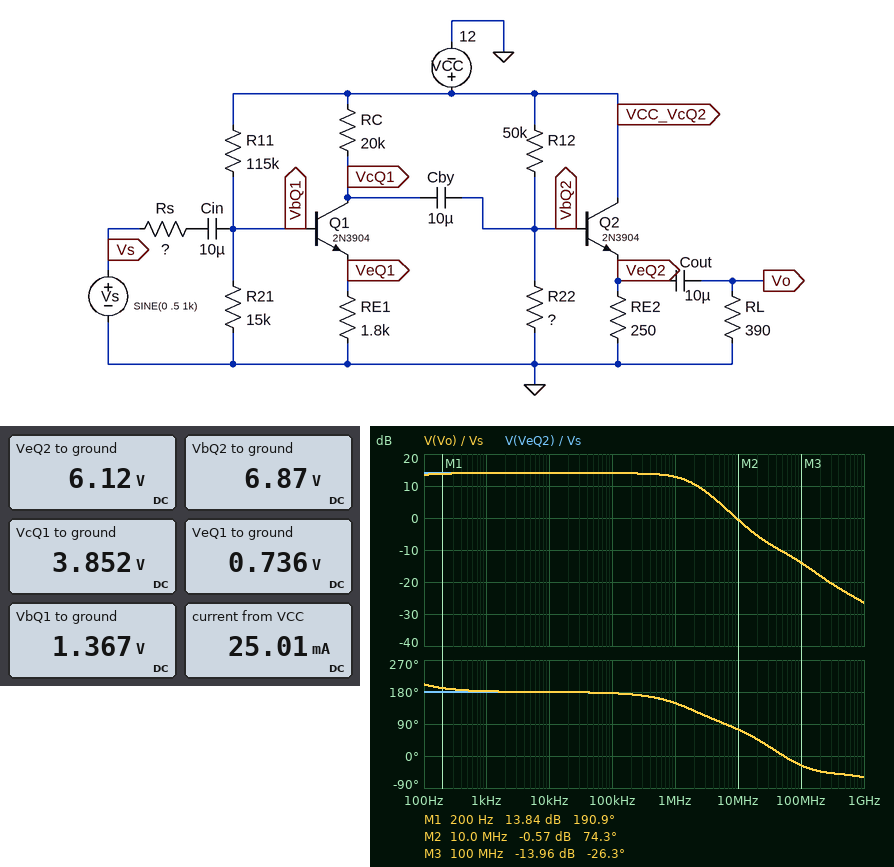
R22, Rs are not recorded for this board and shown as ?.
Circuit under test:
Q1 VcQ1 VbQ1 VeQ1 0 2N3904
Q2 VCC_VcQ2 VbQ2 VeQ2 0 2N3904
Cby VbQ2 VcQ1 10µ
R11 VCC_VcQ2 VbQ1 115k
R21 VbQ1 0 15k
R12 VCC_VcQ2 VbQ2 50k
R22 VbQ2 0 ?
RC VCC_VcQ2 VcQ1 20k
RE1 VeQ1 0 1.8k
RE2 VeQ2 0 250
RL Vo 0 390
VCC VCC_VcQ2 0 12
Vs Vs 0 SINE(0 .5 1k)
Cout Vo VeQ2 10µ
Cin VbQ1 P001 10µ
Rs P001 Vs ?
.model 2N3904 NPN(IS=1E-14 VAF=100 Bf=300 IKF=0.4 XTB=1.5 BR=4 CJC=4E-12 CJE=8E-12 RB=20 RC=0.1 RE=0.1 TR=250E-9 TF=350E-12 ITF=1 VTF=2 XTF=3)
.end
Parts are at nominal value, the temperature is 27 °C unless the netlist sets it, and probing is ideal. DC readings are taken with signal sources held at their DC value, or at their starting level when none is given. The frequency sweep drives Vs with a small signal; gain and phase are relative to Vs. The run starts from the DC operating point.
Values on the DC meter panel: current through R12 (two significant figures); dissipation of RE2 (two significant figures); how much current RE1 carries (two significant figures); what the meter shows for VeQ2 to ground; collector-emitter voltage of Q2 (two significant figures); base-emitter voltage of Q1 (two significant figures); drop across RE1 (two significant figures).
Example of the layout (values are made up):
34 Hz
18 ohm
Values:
100 µA
150 mW
410 µA
6.12 V
5.9 V
630 mV
740 mV
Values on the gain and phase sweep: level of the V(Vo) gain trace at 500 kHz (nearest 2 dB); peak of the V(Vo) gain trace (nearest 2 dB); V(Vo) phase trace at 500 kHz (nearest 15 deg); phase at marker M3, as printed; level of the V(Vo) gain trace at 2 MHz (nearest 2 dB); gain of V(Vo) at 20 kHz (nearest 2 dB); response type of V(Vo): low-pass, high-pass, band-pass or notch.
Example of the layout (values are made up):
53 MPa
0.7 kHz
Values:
14 dB
14 dB
165 deg
-26.3 deg
10 dB
14 dB
low-pass
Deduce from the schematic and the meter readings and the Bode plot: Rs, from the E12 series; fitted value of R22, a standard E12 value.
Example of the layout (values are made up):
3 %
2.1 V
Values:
1.2 kΩ
330 kΩ
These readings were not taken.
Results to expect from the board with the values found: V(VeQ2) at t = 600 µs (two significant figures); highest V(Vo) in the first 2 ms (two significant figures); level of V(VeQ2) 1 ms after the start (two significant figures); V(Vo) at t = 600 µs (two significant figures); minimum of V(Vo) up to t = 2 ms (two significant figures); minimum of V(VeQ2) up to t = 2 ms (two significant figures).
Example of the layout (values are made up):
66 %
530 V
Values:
7.6 V
2.5 V
6.1 V
1.6 V
-2.4 V
3.6 V
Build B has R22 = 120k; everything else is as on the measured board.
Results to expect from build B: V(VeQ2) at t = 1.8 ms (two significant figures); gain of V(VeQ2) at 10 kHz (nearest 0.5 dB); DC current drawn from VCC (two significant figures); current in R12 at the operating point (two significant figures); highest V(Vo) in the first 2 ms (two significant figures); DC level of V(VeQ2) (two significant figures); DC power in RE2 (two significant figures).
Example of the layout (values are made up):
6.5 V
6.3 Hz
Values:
7.5 V
13.5 dB
22 mA
120 µA
2.4 V
5.3 V
110 mW
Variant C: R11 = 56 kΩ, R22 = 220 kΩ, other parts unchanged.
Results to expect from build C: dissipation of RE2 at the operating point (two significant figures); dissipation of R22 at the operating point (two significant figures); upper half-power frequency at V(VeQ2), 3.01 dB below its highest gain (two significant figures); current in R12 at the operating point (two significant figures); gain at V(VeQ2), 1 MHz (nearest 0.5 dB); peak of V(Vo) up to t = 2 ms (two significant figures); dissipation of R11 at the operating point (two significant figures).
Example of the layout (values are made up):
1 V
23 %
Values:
140 mW
200 µW
52 MHz
110 µA
-5.5 dB
1.3 V
1.9 mW
